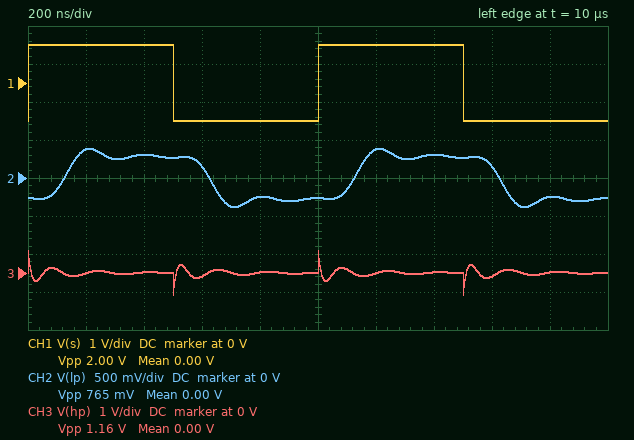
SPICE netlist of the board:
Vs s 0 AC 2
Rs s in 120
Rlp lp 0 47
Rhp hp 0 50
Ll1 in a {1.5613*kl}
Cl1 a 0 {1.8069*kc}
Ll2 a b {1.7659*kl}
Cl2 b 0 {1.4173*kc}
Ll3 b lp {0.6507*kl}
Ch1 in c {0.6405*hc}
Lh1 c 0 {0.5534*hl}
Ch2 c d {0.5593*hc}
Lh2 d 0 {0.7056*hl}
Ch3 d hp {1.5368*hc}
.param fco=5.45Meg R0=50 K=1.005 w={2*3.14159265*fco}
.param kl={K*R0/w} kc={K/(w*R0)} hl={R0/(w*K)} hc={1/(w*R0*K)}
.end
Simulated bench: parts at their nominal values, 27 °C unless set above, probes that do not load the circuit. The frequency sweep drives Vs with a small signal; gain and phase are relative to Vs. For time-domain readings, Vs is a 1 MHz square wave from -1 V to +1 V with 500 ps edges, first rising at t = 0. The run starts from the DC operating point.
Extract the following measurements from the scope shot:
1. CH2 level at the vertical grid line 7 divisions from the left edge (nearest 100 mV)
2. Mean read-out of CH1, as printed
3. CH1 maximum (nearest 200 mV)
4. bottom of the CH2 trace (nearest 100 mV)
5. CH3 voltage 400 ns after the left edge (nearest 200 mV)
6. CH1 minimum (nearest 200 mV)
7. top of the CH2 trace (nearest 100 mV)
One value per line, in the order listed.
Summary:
300 mV
0.00 V
1.0 V
-400 mV
0 V
-1.0 V
400 mV
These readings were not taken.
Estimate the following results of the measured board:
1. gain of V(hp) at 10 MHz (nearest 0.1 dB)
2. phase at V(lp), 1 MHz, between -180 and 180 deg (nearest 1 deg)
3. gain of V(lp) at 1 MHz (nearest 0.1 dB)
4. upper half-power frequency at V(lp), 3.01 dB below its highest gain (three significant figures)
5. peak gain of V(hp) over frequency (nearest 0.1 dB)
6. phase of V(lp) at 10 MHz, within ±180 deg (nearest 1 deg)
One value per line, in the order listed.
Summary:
-10.6 dB
-41 deg
-10.9 dB
5.45 MHz
-10.6 dB
-38 deg
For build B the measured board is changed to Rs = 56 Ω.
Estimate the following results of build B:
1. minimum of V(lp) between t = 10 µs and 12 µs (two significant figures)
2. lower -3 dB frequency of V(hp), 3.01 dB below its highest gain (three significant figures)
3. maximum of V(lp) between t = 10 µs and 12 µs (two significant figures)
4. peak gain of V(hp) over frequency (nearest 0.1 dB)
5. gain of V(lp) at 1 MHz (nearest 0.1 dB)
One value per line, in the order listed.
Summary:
-610 mV
5.45 MHz
610 mV
-6.5 dB
-6.8 dB
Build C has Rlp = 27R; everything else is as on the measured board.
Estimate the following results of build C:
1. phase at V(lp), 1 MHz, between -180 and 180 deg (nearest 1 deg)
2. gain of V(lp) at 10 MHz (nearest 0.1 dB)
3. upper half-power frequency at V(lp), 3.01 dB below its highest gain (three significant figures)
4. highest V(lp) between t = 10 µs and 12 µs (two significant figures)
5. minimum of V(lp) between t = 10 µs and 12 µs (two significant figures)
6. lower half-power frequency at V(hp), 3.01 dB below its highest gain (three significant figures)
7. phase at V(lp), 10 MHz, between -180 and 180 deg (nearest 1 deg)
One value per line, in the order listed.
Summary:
-35 deg
-50.5 dB
5.29 MHz
300 mV
-300 mV
5.25 MHz
-54 deg
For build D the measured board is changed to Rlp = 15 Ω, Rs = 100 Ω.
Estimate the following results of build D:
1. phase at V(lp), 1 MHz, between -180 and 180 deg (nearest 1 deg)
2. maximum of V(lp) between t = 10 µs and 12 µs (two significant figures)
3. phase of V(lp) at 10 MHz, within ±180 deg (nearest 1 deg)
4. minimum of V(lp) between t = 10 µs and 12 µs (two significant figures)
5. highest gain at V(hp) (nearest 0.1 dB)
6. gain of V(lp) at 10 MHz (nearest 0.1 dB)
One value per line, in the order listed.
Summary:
-32 deg
230 mV
-68 deg
-230 mV
-9.5 dB
-53.3 dB
